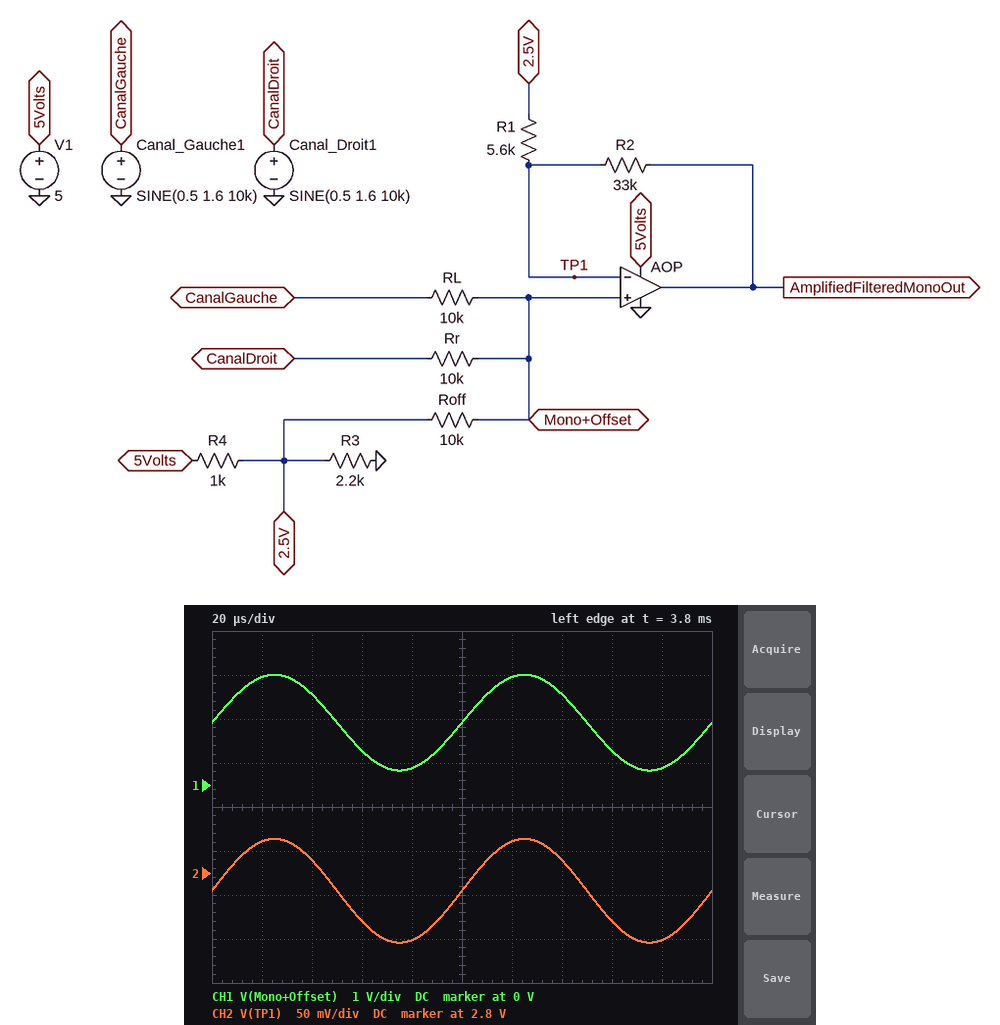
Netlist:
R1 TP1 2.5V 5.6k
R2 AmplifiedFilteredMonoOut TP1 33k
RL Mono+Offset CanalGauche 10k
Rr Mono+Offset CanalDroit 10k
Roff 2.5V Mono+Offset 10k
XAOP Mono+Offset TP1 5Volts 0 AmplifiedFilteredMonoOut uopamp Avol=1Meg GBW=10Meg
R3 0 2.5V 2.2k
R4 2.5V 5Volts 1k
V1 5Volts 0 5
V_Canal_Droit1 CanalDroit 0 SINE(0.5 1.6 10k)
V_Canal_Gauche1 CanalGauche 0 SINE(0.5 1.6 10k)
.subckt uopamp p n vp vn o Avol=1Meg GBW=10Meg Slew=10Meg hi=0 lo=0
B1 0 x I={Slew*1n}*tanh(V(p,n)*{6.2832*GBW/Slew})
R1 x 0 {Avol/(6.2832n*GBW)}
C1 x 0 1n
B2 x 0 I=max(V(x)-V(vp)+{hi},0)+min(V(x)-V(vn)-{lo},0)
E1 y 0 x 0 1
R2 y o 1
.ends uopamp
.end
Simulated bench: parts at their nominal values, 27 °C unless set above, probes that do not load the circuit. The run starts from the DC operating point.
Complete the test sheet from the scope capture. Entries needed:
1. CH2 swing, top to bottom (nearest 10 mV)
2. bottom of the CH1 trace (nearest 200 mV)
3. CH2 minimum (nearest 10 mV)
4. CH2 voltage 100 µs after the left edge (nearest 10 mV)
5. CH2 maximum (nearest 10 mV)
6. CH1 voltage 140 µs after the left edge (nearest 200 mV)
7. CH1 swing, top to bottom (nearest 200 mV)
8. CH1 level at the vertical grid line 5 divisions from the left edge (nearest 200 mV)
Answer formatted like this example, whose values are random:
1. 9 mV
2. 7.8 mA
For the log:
1. 120 mV
2. 400 mV
3. 2.72 V
4. 2.78 V
5. 2.84 V
6. 2.0 V
7. 2.2 V
8. 1.4 V
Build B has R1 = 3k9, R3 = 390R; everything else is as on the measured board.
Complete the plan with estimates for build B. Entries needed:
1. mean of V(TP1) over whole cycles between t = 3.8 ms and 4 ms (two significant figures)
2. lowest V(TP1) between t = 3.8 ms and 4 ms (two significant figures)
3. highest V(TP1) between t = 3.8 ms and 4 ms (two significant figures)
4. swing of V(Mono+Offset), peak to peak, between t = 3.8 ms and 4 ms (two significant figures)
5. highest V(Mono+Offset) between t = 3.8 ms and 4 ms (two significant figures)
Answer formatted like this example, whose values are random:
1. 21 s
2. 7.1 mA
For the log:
1. 1.4 V
2. 1.2 V
3. 1.8 V
4. 2.2 V
5. 1.9 V
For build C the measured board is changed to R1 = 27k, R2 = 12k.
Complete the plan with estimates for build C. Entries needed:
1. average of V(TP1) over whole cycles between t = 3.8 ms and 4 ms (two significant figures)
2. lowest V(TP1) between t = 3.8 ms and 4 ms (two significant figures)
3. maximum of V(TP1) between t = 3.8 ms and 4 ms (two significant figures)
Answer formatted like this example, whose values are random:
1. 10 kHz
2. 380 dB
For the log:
1. 1.6 V
2. 970 mV
3. 2.5 V
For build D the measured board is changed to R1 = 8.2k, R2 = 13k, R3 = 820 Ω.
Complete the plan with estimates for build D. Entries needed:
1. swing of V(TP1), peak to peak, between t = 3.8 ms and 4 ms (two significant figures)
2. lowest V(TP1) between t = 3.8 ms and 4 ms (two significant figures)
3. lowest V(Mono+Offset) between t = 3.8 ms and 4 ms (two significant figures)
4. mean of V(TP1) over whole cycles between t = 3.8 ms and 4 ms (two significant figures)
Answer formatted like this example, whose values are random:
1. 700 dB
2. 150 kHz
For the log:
1. 860 mV
2. 1.3 V
3. -30 mV
4. 1.5 V
